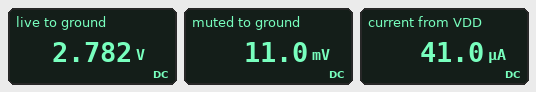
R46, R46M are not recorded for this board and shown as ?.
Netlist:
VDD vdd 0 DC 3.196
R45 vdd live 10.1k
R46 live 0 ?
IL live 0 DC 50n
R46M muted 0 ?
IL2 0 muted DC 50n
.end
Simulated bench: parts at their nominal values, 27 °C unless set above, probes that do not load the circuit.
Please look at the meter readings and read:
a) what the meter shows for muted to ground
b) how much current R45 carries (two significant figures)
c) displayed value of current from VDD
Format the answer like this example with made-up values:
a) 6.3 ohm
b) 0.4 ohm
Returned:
a) 11.0 mV
b) 41 µA
c) 41.0 µA
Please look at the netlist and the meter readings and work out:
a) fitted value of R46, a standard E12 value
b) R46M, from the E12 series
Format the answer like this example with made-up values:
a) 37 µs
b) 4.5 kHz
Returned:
a) 68 kΩ
b) 220 kΩ
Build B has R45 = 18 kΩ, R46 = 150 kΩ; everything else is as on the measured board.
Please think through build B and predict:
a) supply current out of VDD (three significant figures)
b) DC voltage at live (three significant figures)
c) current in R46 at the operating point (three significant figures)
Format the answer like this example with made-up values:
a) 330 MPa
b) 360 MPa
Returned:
a) 19.1 µA
b) 2.85 V
c) 19.0 µA
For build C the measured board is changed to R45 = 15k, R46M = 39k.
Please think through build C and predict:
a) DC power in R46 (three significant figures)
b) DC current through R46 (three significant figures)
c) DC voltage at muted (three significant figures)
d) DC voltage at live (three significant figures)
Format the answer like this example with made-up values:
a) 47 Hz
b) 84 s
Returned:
a) 101 µW
b) 38.5 µA
c) 1.95 mV
d) 2.62 V
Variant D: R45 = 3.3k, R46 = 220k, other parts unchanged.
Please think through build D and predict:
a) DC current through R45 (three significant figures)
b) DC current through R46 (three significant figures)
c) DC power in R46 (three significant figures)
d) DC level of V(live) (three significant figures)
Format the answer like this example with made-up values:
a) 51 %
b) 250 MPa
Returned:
a) 14.4 µA
b) 14.3 µA
c) 45.1 µW
d) 3.15 V
